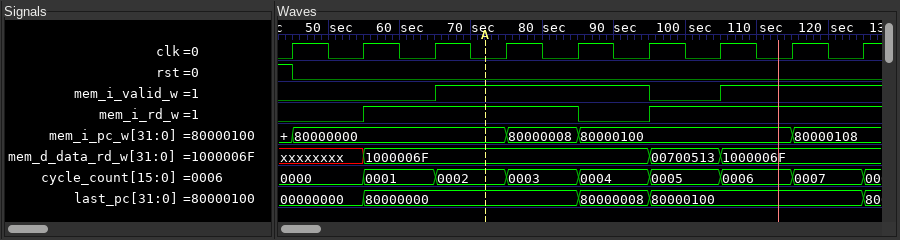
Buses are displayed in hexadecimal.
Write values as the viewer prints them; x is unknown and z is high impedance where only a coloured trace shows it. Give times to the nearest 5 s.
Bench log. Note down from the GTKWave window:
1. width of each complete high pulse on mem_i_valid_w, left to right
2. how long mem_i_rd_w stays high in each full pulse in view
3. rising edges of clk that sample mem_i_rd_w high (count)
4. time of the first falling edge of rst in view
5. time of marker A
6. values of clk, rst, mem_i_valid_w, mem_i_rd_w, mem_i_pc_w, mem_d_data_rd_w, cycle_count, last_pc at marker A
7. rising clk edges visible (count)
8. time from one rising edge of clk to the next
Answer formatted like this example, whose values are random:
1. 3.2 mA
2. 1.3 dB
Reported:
1. 30 s
2. 30 s
3. 6
4. 45 s
5. 70 s
6. clk=0, rst=0, mem_i_valid_w=1, mem_i_rd_w=1, mem_i_pc_w=80000000, mem_d_data_rd_w=1000006F, cycle_count=0002, last_pc=80000000
7. 9
8. 10 s
